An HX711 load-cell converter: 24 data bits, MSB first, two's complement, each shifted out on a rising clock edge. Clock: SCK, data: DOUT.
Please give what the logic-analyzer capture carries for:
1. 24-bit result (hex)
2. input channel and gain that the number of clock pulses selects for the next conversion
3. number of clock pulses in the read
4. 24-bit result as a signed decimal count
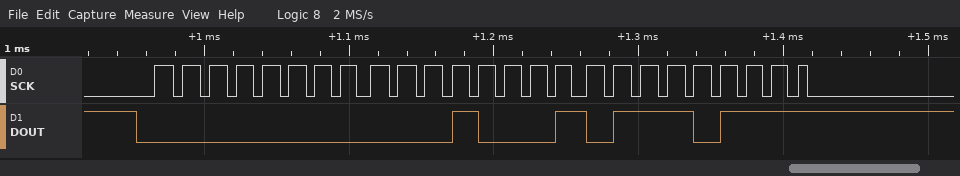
0x001177
channel A, gain 128
25
4471
